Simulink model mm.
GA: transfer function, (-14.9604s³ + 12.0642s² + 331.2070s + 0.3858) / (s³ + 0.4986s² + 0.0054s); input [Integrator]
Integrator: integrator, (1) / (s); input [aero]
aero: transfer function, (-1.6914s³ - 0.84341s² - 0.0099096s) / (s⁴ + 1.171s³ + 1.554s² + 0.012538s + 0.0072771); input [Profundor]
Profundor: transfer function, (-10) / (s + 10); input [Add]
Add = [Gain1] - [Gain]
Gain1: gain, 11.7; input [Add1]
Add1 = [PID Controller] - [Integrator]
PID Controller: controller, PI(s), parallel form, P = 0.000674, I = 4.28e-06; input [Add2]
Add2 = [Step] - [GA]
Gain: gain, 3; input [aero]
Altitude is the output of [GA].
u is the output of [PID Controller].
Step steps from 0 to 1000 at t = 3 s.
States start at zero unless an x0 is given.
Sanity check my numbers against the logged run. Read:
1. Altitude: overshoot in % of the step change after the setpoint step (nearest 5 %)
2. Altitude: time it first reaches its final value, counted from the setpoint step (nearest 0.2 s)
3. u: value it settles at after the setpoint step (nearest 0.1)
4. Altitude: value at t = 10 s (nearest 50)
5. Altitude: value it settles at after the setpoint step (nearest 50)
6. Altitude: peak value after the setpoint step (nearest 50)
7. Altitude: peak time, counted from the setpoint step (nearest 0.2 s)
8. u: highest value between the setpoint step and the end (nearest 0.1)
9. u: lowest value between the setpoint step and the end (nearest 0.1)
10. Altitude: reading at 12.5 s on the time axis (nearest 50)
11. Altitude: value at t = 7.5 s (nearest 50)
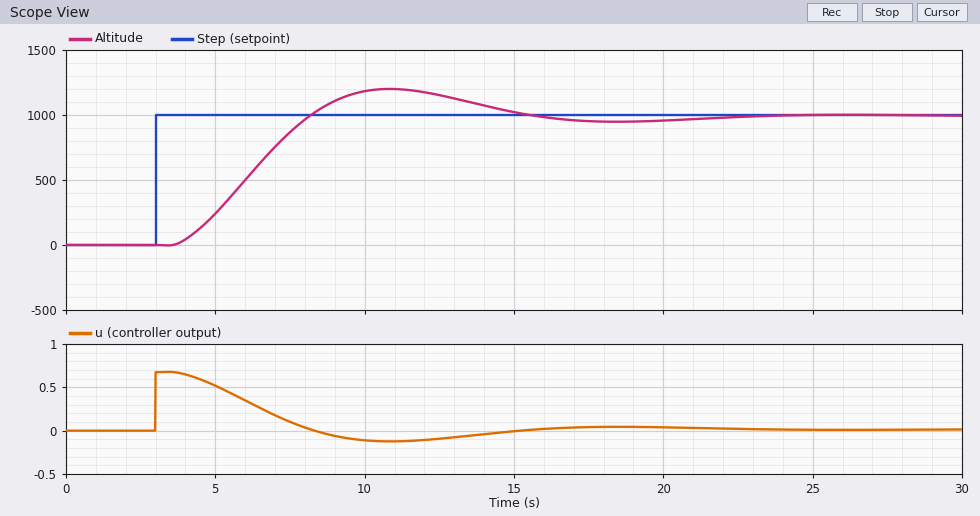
20 %
5.2 s
0.0
1200
1000
1200
7.8 s
0.7
-0.1
1150
850
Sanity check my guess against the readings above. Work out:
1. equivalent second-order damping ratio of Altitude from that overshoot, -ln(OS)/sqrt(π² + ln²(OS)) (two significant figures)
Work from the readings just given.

0.46
